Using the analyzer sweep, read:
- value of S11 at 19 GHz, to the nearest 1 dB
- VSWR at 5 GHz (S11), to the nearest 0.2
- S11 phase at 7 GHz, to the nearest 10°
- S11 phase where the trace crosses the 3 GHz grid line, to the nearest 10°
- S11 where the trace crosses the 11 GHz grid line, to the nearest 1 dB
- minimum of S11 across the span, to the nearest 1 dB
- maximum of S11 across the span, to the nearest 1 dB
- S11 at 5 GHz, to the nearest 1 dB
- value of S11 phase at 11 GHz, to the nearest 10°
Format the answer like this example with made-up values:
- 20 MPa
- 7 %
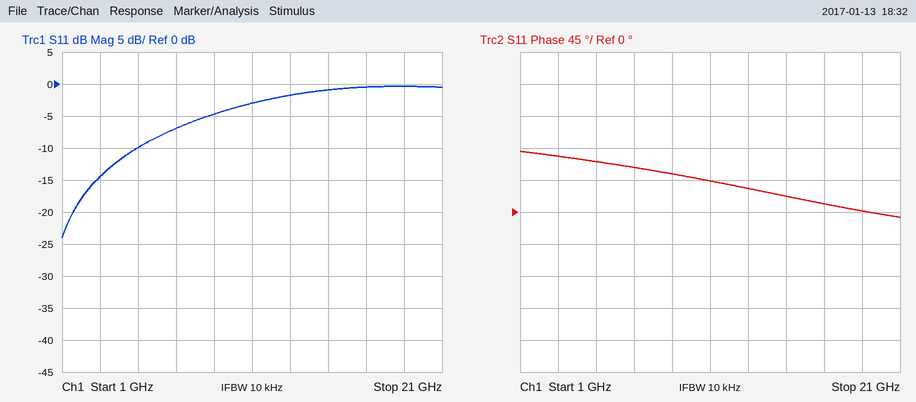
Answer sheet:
- 0 dB
- 2.0
- 60°
- 80°
- -3 dB
- -24 dB
- 0 dB
- -10 dB
- 40°
